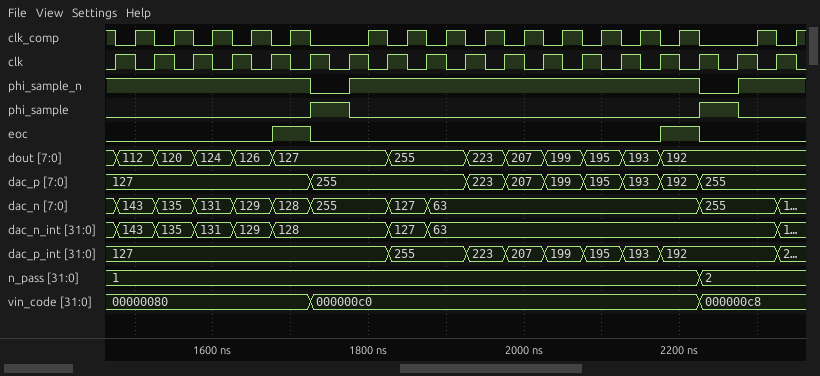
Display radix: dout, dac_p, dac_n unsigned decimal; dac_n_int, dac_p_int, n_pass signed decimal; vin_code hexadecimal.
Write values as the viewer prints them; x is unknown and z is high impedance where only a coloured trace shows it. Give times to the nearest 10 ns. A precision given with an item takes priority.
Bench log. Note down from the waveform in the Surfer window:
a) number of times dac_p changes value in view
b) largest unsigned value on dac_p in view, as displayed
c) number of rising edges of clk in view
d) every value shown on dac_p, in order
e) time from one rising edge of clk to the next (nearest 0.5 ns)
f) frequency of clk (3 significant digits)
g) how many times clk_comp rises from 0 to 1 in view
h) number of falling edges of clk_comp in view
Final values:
8
255
18
127, 255, 223, 207, 199, 195, 193, 192, 255
50 ns
20.0 MHz
16
16
